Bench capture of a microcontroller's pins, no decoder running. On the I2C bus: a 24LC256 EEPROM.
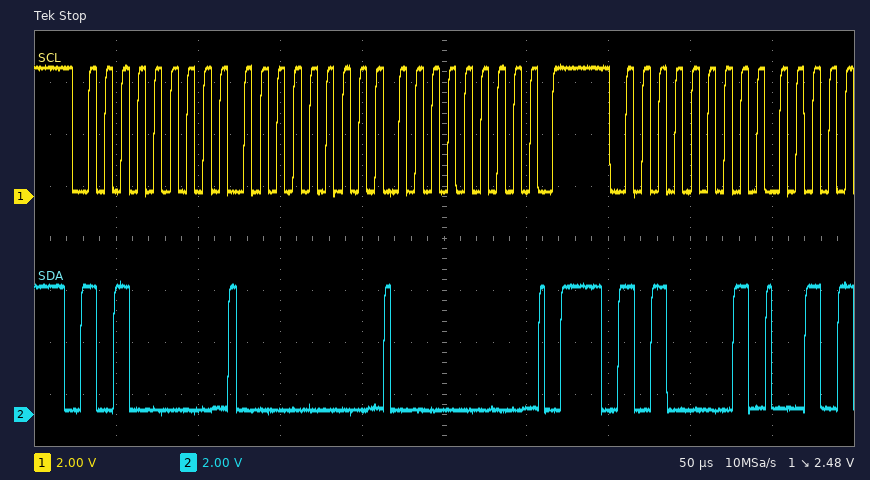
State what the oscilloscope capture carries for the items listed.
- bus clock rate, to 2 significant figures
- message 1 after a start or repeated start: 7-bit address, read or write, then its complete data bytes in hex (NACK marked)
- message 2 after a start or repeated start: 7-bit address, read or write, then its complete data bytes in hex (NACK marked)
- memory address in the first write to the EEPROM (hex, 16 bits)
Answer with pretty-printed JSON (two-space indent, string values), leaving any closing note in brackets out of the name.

{
  "bus clock rate, to 2 significant figures": "100 kHz",
  "message 1 after a start or repeated start: 7-bit address, read or write, then its complete data bytes in hex": "0x50 write: 00 00",
  "message 2 after a start or repeated start: 7-bit address, read or write, then its complete data bytes in hex": "0x50 read",
  "memory address in the first write to the EEPROM": "0x0000"
}
